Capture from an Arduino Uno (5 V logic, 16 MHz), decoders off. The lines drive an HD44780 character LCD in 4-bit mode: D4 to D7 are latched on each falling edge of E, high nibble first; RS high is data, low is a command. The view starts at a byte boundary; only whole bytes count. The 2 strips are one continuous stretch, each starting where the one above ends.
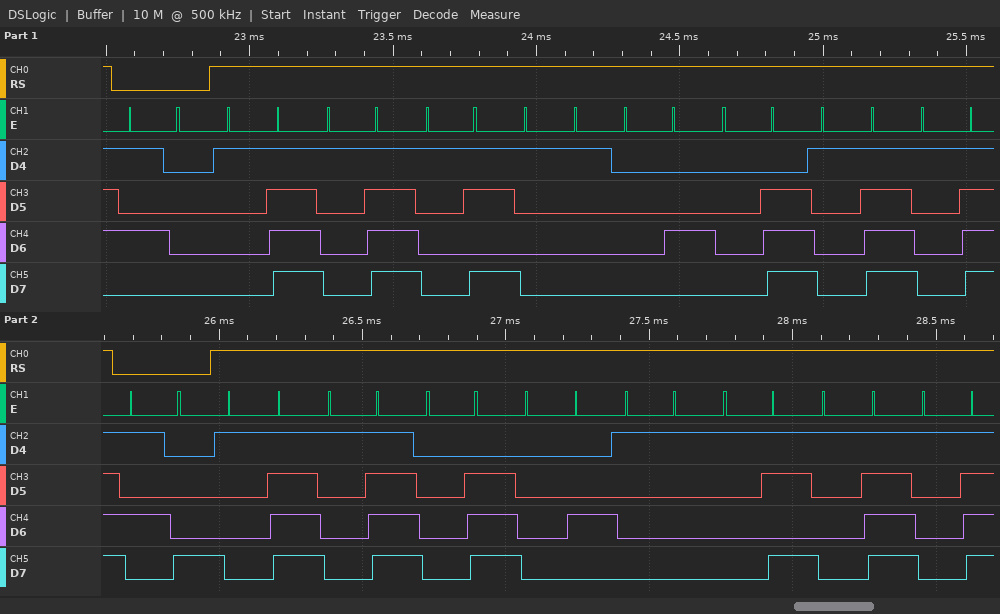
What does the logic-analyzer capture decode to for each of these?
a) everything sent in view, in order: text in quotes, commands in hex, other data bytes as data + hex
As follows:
0x50 data 1F 1F 1B 11 04 0E 1F 1F 0x58 data 1F 1F 0E 04 11 1B 1F 1F
